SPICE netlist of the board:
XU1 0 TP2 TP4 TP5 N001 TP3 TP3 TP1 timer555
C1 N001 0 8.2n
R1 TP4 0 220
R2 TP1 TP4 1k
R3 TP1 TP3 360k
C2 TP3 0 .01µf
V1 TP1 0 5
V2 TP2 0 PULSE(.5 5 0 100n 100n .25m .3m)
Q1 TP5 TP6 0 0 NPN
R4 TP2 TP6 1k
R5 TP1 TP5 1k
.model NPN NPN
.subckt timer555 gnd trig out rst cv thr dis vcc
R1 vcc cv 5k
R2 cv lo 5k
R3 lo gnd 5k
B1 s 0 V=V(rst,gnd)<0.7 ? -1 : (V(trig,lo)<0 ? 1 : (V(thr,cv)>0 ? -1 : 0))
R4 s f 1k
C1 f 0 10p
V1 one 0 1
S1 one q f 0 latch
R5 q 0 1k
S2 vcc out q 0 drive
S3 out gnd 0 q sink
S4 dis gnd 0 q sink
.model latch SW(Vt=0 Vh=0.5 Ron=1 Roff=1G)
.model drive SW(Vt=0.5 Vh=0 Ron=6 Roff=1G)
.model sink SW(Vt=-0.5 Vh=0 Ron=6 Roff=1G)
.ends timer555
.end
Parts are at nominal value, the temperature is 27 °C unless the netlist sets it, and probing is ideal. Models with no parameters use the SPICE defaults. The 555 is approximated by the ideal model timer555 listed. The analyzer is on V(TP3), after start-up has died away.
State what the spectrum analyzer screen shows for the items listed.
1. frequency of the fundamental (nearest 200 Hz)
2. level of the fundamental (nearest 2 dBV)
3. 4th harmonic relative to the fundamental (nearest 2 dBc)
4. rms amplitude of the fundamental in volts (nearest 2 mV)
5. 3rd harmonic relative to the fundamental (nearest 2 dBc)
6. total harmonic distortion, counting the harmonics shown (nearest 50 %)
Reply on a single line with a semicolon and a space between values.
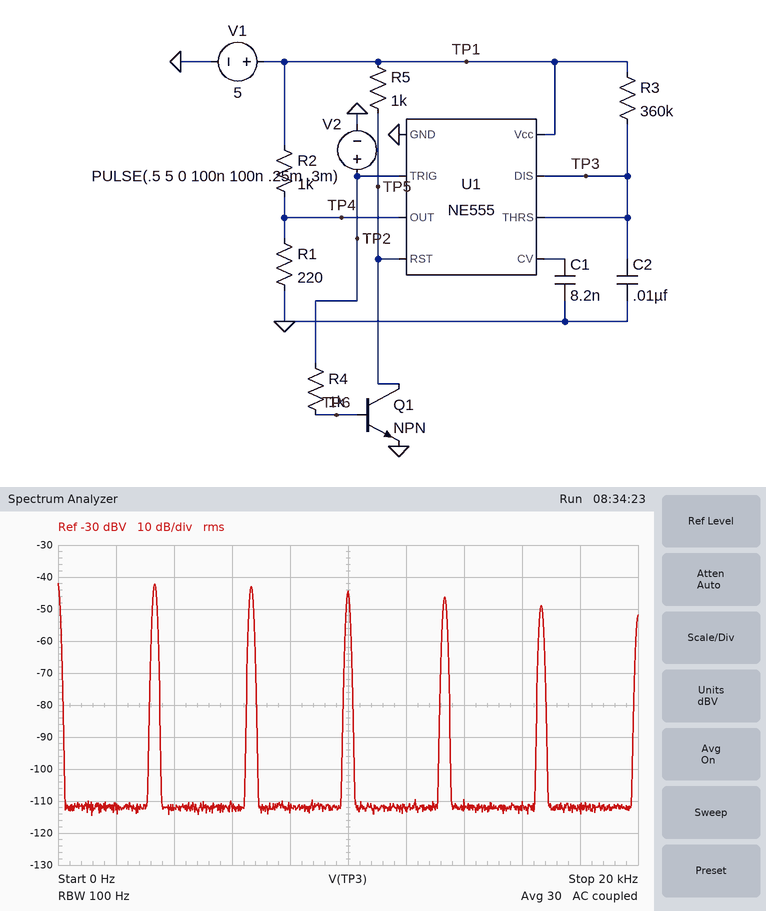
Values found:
3.4 kHz; -42 dBV; -4 dBc; 8 mV; -2 dBc; 150 %
